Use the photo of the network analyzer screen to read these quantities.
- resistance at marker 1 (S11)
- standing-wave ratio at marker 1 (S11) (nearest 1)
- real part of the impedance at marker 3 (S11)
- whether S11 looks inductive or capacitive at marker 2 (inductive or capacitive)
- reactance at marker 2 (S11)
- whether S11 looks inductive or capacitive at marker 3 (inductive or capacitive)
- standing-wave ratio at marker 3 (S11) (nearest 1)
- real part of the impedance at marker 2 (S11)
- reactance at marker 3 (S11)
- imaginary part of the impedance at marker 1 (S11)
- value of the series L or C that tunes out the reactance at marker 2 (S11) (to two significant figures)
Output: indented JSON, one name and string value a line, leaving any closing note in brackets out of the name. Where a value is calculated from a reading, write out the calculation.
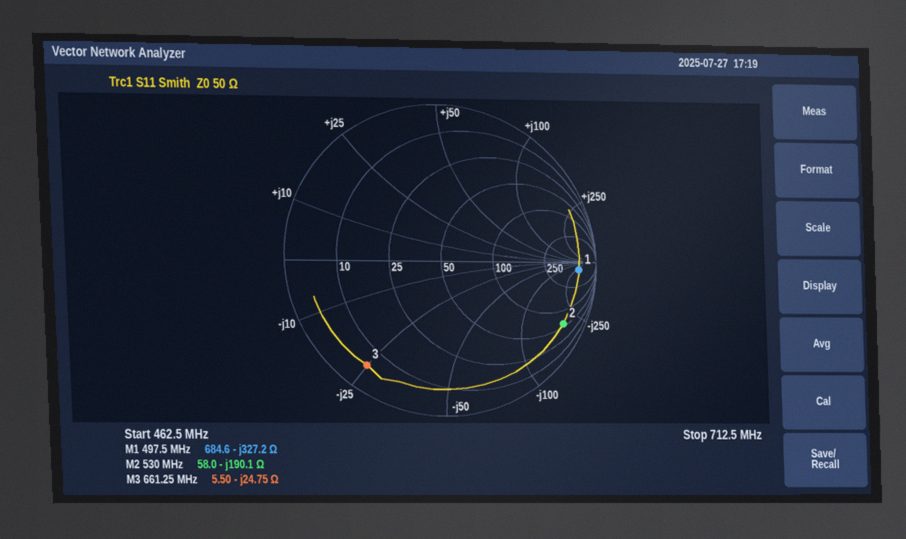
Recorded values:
{
  "resistance at marker 1": "684.6 Ω",
  "standing-wave ratio at marker 1 (S11)": "17",
  "real part of the impedance at marker 3": "5.50 Ω",
  "whether S11 looks inductive or capacitive at marker 2": "capacitive",
  "reactance at marker 2": "-190.1 Ω",
  "whether S11 looks inductive or capacitive at marker 3": "capacitive",
  "standing-wave ratio at marker 3 (S11)": "11",
  "real part of the impedance at marker 2": "58.0 Ω",
  "reactance at marker 3": "-24.75 Ω",
  "imaginary part of the impedance at marker 1": "-327.2 Ω",
  "value of the series L or C that tunes out the reactance at marker 2 (S11)": "L = 190.1 Ω/(2π × 530 MHz) ≈ 57 nH"
}
